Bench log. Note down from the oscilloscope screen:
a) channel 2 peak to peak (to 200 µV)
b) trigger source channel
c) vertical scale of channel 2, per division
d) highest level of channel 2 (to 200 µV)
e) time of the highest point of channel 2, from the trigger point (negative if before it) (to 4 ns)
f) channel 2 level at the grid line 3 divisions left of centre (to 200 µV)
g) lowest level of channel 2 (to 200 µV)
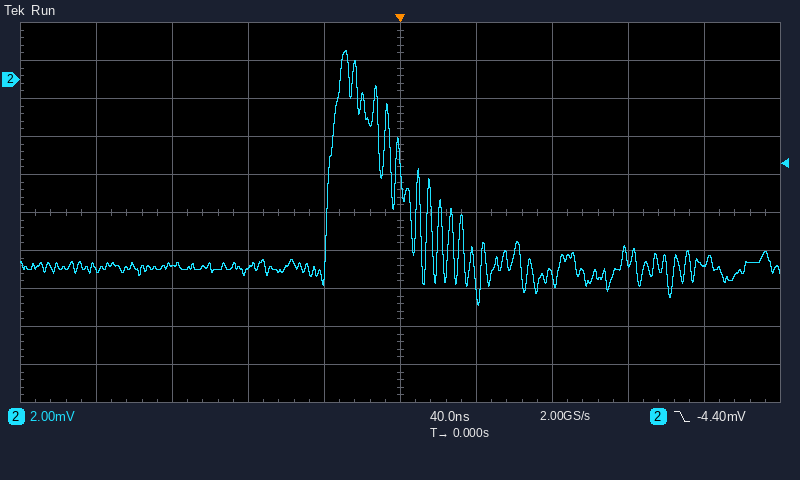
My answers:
13.4 mV
channel 2
2 mV
1.6 mV
-28 ns
-9.8 mV
-11.8 mV
